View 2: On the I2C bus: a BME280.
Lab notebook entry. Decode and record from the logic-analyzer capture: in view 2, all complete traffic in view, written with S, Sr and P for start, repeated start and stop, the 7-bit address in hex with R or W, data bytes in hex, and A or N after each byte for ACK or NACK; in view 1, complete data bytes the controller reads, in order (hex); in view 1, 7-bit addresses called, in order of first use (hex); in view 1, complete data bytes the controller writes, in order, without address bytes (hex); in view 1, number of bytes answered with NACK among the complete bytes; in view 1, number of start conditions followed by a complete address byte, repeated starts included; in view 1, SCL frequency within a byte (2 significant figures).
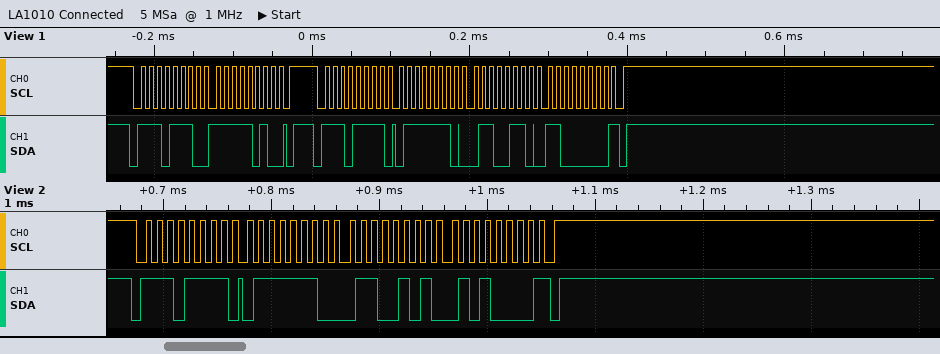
S 77R A 7E A 65 A 50 N P
7E 66 C0
0x77
FA
1
2
100 kHz
